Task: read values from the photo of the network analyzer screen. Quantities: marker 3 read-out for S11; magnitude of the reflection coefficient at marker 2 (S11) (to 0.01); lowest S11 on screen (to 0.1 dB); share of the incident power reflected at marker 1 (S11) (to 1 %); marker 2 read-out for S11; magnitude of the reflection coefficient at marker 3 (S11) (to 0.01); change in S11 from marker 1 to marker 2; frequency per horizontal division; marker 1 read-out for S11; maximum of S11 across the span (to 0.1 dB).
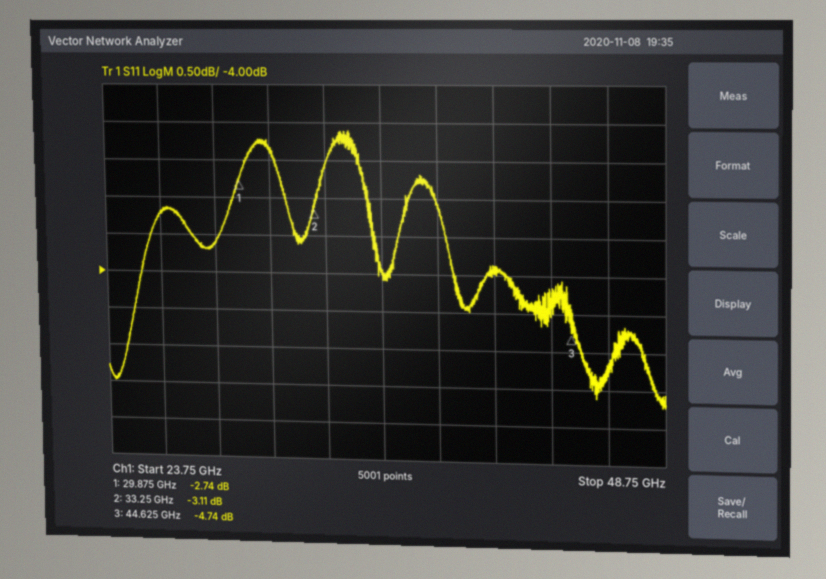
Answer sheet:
-4.74 dB
0.70
-5.7 dB
53 %
-3.11 dB
0.58
-0.37 dB
2.5 GHz
-2.74 dB
-2.1 dB
